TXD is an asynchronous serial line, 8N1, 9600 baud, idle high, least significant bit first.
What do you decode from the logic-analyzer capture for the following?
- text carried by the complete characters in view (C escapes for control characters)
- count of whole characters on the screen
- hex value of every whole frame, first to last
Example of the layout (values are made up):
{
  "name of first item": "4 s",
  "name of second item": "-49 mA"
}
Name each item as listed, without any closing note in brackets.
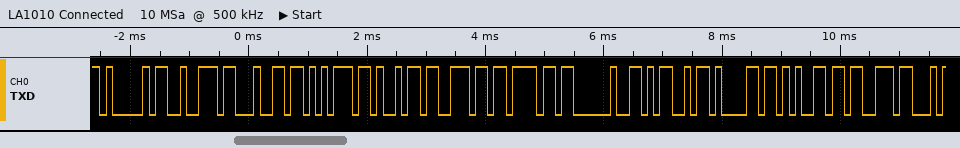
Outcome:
{
  "text carried by the complete characters in view": "\"Arduino Maes\"",
  "count of whole characters on the screen": "12",
  "hex value of every whole frame, first to last": "41 72 64 75 69 6E 6F 20 4D 61 65 73"
}
